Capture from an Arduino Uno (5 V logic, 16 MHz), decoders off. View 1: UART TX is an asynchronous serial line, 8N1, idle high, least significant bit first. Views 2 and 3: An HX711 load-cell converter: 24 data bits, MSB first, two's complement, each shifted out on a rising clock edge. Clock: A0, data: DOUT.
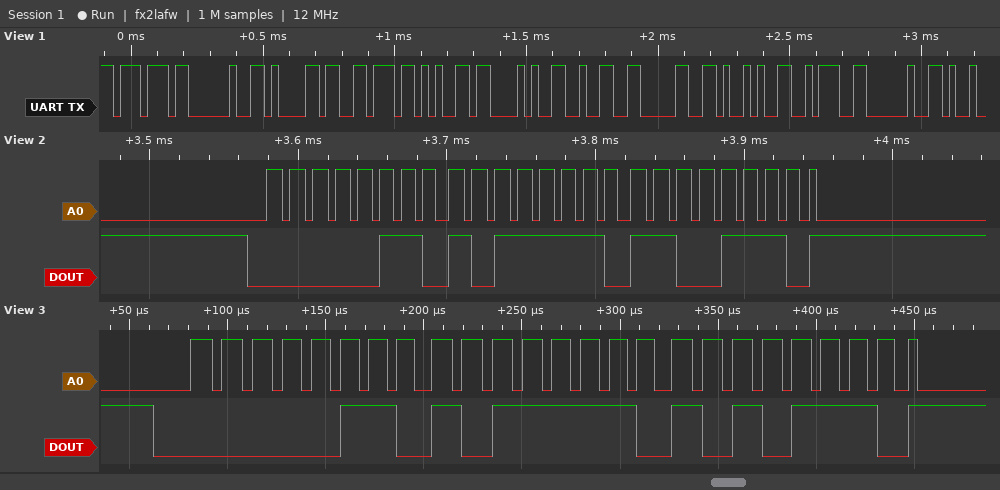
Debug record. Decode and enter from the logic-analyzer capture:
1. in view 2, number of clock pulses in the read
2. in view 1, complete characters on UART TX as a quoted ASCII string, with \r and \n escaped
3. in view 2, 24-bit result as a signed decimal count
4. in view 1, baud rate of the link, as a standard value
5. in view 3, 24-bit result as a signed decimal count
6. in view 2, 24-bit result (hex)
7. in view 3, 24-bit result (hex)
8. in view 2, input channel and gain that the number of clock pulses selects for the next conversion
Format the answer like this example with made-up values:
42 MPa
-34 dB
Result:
25
"w ave(20): "
442062
38400 baud
442030
0x06BECE
0x06BEAE
channel A, gain 128
